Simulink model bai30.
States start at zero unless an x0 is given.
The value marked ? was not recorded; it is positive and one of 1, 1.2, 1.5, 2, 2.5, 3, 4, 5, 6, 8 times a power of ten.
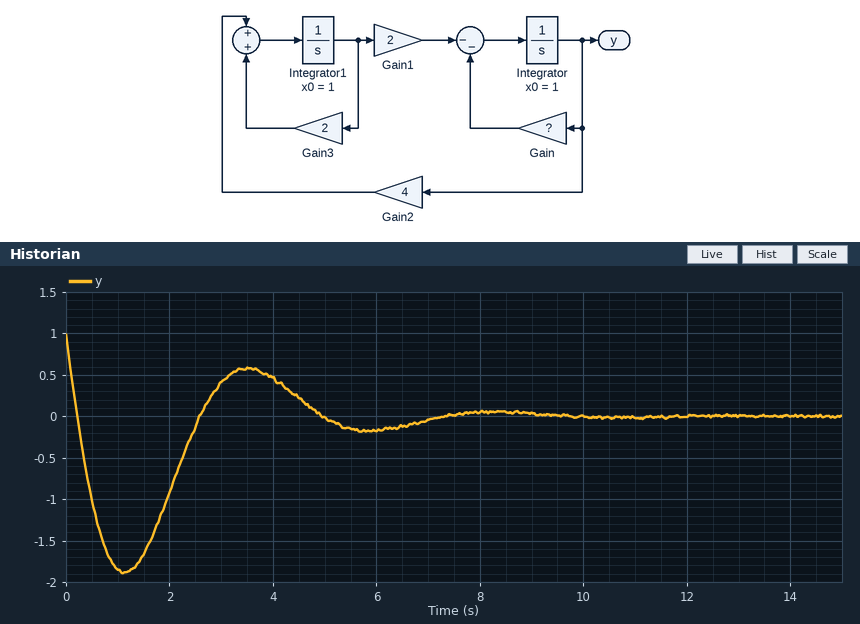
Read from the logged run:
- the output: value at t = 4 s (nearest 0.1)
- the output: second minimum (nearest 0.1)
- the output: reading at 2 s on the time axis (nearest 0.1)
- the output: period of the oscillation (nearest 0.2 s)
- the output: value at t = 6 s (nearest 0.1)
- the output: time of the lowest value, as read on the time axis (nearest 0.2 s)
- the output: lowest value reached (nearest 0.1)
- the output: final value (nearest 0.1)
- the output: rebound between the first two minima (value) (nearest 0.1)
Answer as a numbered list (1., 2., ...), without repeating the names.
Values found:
1. 0.5
2. -0.2
3. -0.9
4. 4.8 s
5. -0.2
6. 1.2 s
7. -1.9
8. 0.0
9. 0.6
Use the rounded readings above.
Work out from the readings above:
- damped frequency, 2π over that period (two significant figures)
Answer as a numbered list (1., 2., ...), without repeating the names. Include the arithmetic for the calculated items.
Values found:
1. 2π / 4.8 = 1.3 rad/s
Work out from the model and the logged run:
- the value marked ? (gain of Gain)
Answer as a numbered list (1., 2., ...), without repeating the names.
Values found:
1. 3
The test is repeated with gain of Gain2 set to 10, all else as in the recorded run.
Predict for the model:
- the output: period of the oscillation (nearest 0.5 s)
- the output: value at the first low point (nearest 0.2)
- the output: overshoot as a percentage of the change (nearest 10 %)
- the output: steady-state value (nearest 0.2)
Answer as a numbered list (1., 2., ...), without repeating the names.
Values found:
1. 1.5 s
2. -1.2
3. 120 %
4. 0.0
